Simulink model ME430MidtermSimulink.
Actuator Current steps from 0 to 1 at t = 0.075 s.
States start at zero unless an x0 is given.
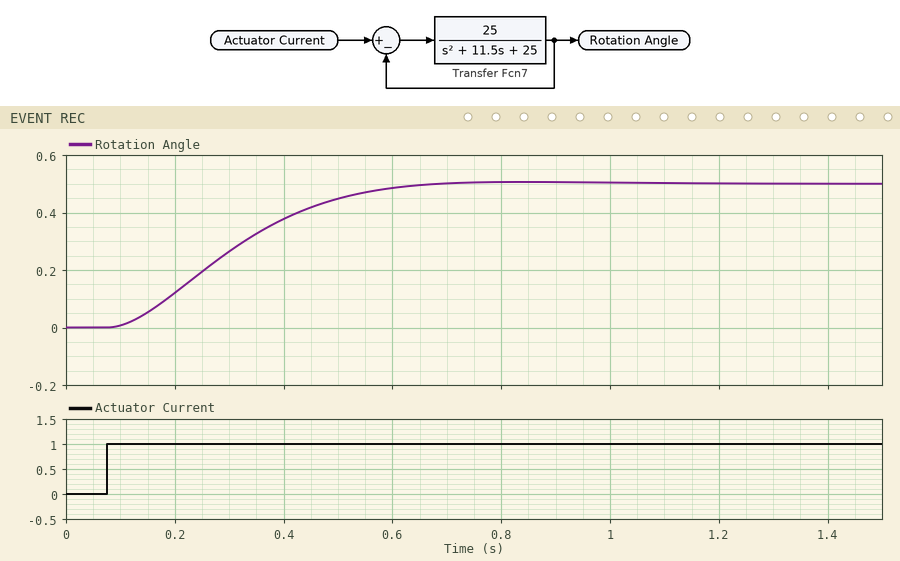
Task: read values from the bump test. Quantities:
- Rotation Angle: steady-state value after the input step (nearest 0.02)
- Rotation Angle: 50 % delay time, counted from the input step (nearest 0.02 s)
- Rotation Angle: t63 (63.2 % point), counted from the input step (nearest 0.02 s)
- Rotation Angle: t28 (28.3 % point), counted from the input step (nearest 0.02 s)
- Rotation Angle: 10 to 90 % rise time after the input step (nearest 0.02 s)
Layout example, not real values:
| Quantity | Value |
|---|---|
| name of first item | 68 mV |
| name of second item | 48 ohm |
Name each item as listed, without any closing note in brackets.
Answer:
| Quantity | Value |
|---|---|
| Rotation Angle: steady-state value after the input step | 0.50 |
| Rotation Angle: 50 % delay time, counted from the input step | 0.22 s |
| Rotation Angle: t63 (63.2 % point), counted from the input step | 0.26 s |
| Rotation Angle: t28 (28.3 % point), counted from the input step | 0.14 s |
| Rotation Angle: 10 to 90 % rise time after the input step | 0.36 s |
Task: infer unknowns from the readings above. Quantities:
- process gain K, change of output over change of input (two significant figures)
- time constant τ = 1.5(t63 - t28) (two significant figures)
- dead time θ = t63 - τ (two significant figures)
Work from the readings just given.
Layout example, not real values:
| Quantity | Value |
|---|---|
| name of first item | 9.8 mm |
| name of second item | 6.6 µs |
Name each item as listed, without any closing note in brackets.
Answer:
| Quantity | Value |
|---|---|
| process gain K, change of output over change of input | 0.50 |
| time constant τ = 1.5(t63 - t28) | 0.18 s |
| dead time θ = t63 - τ | 0.080 s |
